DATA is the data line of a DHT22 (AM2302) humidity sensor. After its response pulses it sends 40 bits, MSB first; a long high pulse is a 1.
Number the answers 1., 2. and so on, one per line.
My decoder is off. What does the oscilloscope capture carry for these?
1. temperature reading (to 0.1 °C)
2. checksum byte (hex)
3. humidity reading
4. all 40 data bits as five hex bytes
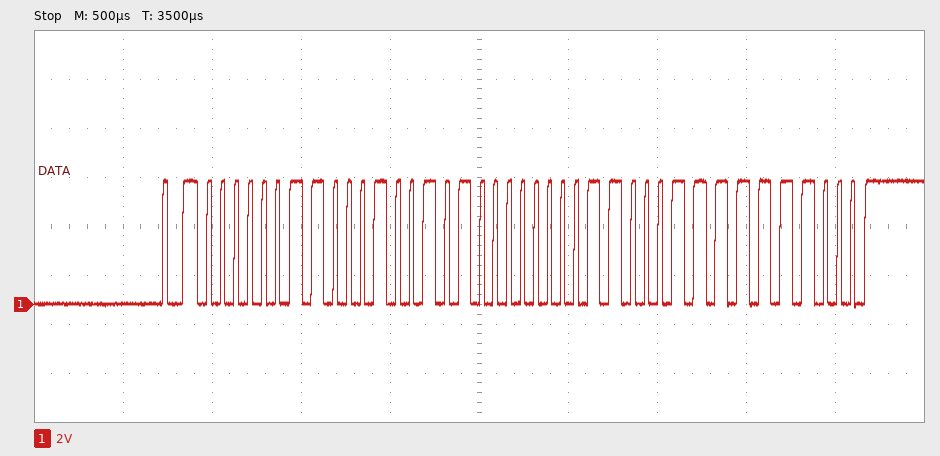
1. -9.9 °C
2. 0xF8
3. 78.6 %
4. 03 12 80 63 F8
